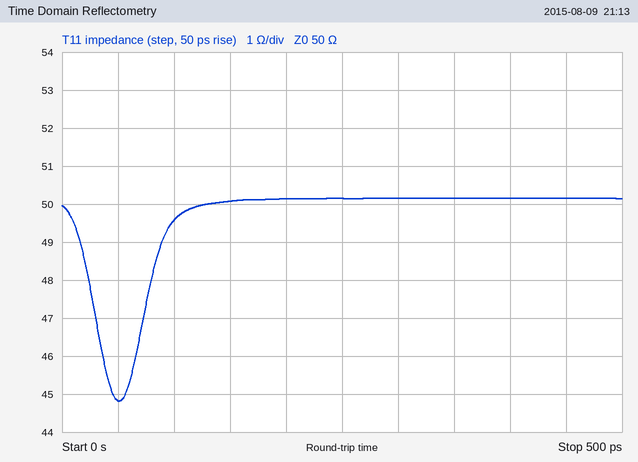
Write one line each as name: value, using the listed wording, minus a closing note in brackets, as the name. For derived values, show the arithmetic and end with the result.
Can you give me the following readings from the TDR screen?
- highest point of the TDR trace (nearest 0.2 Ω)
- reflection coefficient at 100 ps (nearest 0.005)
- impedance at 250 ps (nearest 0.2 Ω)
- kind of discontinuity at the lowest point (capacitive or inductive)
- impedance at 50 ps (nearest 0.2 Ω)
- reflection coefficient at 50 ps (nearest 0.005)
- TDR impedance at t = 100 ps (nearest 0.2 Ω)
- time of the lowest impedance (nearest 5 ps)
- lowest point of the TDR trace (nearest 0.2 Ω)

highest point of the TDR trace: 50.2 Ω
reflection coefficient at 100 ps: (49.6 − 50)/(49.6 + 50) ≈ -0.00402, so -0.005 to the nearest 0.005
impedance at 250 ps: 50.2 Ω
kind of discontinuity at the lowest point: capacitive
impedance at 50 ps: 44.8 Ω
reflection coefficient at 50 ps: (44.8 − 50)/(44.8 + 50) ≈ -0.055
TDR impedance at t = 100 ps: 49.6 Ω
time of the lowest impedance: 50 ps
lowest point of the TDR trace: 44.8 Ω
